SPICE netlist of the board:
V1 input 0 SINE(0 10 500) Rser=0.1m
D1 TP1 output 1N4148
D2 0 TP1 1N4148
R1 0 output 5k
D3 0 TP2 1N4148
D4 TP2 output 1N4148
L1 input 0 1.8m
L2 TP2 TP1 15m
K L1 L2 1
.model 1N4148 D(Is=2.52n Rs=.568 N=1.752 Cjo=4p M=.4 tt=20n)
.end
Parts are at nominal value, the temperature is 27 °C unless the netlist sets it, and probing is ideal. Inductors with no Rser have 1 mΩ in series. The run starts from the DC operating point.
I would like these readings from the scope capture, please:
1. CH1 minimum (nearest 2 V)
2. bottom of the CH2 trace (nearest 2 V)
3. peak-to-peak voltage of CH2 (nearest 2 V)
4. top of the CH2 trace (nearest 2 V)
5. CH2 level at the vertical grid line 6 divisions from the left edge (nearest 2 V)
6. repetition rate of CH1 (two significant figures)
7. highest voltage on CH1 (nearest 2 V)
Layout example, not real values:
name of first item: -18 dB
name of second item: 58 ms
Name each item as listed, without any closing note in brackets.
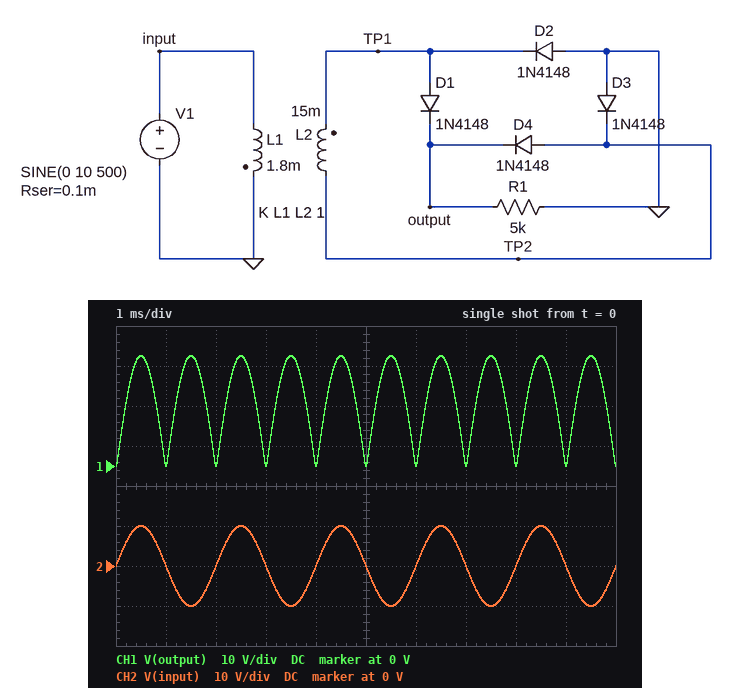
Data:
CH1 minimum: 0 V
bottom of the CH2 trace: -10 V
peak-to-peak voltage of CH2: 20 V
top of the CH2 trace: 10 V
CH2 level at the vertical grid line 6 divisions from the left edge: 0 V
repetition rate of CH1: 1.0 kHz
highest voltage on CH1: 28 V
